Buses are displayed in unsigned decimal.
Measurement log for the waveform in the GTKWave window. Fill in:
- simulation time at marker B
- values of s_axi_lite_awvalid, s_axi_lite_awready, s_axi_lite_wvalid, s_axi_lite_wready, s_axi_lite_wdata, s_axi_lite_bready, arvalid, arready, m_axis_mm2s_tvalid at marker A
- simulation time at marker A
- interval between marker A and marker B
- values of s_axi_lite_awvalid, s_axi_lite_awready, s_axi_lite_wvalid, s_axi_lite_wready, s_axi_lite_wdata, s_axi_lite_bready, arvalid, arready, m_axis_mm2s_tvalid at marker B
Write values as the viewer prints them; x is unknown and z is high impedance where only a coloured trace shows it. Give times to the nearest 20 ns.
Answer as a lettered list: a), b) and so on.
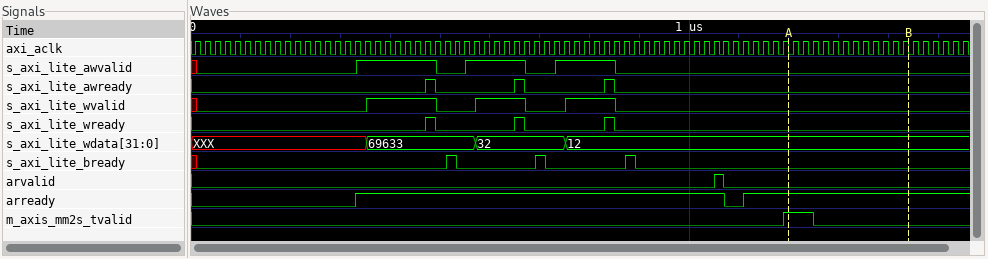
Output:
a) 1440 ns
b) s_axi_lite_awvalid=0, s_axi_lite_awready=0, s_axi_lite_wvalid=0, s_axi_lite_wready=0, s_axi_lite_wdata=12, s_axi_lite_bready=0, arvalid=0, arready=1, m_axis_mm2s_tvalid=1
c) 1200 ns
d) 240 ns
e) s_axi_lite_awvalid=0, s_axi_lite_awready=0, s_axi_lite_wvalid=0, s_axi_lite_wready=0, s_axi_lite_wdata=12, s_axi_lite_bready=0, arvalid=0, arready=1, m_axis_mm2s_tvalid=0
